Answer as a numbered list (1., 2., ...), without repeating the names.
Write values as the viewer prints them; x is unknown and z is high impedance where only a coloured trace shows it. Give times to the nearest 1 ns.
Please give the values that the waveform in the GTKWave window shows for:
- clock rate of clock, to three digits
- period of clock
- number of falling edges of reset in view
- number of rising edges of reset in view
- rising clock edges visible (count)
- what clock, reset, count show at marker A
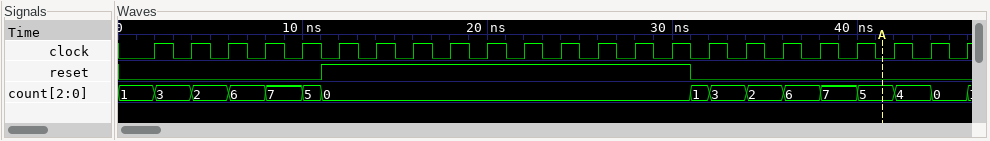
1. 500 MHz
2. 2 ns
3. 1
4. 1
5. 23
6. clock=0, reset=0, count=5
